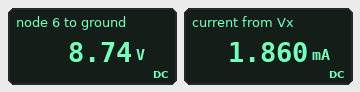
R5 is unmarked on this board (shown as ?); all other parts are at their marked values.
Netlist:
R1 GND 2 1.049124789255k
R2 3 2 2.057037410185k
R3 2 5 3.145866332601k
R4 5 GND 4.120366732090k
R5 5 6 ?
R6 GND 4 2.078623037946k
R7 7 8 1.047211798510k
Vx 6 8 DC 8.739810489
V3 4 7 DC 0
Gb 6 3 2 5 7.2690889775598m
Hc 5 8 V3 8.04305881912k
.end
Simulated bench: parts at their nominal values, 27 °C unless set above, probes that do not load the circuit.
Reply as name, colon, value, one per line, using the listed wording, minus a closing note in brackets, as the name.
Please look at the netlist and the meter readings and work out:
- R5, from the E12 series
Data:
R5, from the E12 series: 4.7 kΩ
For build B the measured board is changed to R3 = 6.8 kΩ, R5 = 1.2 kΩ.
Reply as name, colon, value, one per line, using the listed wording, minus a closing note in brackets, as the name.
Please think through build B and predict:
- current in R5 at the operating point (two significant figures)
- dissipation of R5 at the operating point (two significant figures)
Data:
current in R5 at the operating point: 7.3 mA
dissipation of R5 at the operating point: 64 mW
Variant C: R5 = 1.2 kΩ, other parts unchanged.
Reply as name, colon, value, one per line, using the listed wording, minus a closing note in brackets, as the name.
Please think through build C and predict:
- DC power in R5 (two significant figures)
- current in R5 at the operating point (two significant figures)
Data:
DC power in R5: 64 mW
current in R5 at the operating point: 7.3 mA
